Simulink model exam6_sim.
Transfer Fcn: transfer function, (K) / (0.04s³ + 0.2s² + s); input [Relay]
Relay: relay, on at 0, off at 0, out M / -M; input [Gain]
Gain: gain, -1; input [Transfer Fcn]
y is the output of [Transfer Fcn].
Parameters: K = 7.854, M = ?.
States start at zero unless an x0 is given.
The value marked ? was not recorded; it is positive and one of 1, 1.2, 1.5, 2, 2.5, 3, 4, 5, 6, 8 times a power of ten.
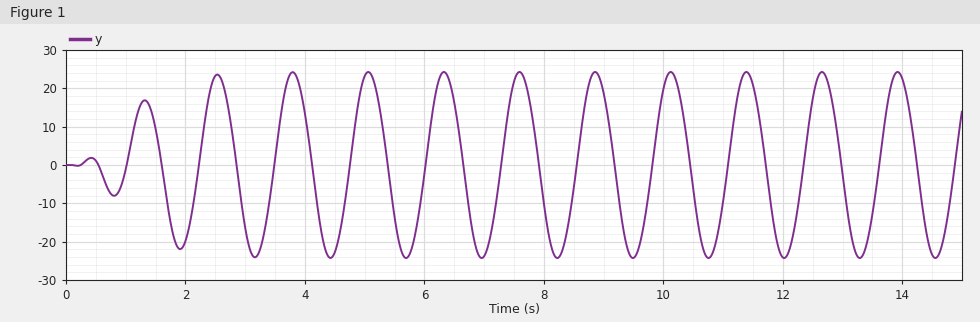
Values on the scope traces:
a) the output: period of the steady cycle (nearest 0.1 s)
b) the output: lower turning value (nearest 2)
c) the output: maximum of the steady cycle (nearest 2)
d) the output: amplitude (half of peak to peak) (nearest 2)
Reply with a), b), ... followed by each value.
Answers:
a) 1.3 s
b) -24
c) 24
d) 24
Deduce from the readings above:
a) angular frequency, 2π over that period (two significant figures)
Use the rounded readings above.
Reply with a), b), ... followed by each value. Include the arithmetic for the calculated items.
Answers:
a) 2π / 1.3 = 4.8 rad/s
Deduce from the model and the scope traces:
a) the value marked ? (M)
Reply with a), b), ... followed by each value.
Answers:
a) 12
